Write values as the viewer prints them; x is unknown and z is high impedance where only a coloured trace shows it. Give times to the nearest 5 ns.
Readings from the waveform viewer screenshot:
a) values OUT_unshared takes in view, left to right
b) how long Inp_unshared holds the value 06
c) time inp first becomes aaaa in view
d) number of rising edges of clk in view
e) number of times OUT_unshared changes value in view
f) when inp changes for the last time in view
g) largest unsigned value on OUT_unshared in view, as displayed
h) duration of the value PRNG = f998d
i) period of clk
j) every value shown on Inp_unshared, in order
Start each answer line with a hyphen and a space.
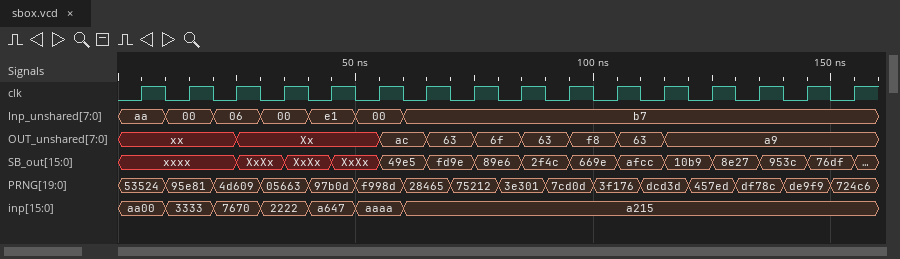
- xx, Xx, ac, 63, 6f, 63, f8, 63, a9
- 10 ns
- 50 ns
- 16
- 8
- 60 ns
- f8
- 10 ns
- 10 ns
- aa, 00, 06, 00, e1, 00, b7
